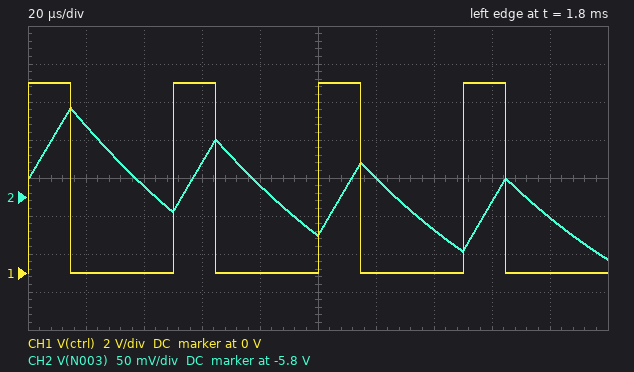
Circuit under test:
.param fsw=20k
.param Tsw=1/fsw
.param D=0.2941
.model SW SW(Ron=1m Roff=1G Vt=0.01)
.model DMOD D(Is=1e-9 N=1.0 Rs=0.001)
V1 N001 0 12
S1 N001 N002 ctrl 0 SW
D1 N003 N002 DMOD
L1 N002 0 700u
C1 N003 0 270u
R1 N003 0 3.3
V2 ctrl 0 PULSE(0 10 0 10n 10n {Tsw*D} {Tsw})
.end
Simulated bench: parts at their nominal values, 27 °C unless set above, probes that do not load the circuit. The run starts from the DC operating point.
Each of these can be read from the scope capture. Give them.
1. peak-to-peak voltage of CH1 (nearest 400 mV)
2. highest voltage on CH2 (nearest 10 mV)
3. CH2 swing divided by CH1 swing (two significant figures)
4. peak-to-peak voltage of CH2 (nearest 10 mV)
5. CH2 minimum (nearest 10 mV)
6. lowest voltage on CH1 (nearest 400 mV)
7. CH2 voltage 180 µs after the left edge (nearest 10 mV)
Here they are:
10.0 V
-5.68 V
0.020
200 mV
-5.88 V
0 V
-5.83 V
